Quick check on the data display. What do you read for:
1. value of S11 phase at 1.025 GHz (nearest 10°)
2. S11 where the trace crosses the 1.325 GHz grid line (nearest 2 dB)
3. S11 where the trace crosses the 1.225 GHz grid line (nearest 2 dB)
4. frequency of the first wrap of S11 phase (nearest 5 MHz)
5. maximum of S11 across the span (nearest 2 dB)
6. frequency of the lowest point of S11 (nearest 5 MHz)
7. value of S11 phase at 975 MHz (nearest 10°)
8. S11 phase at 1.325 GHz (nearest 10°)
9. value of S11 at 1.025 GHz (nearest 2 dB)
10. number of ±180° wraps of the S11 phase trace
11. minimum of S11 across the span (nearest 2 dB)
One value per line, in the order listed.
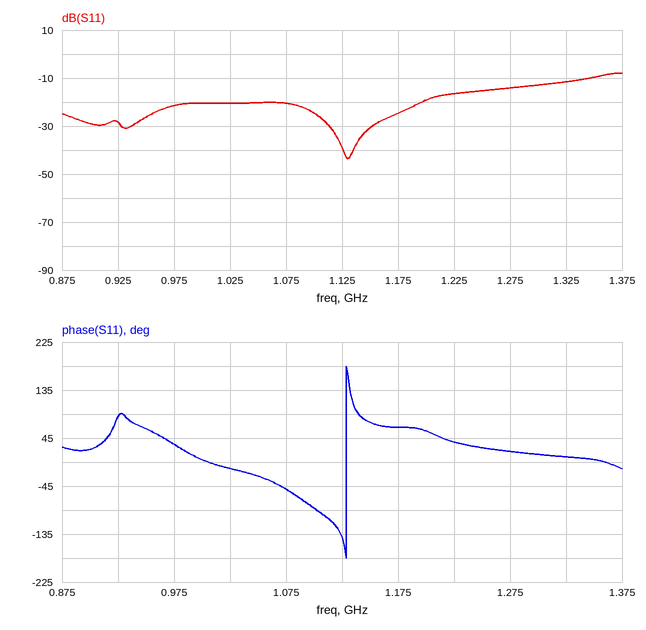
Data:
-10°
-12 dB
-16 dB
1.130 GHz
-8 dB
1.130 GHz
30°
10°
-20 dB
1
-44 dB
